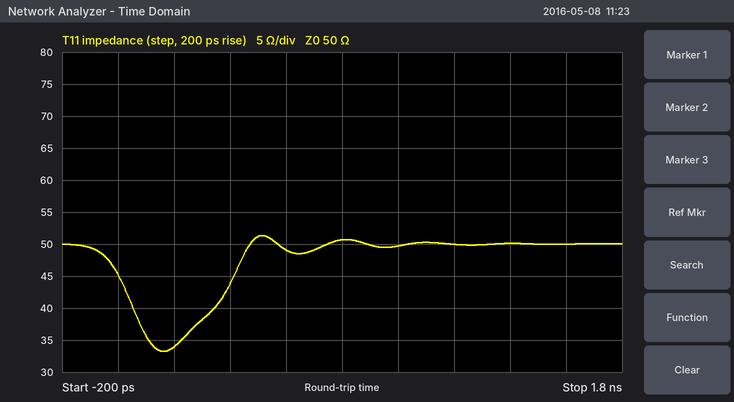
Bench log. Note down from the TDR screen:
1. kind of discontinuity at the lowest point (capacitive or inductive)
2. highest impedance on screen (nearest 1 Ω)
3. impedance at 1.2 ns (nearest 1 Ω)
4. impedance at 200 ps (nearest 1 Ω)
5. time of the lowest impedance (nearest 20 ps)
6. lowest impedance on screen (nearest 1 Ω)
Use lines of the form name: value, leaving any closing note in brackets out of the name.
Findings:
kind of discontinuity at the lowest point: capacitive
highest impedance on screen: 51 Ω
impedance at 1.2 ns: 50 Ω
impedance at 200 ps: 34 Ω
time of the lowest impedance: 160 ps
lowest impedance on screen: 33 Ω
